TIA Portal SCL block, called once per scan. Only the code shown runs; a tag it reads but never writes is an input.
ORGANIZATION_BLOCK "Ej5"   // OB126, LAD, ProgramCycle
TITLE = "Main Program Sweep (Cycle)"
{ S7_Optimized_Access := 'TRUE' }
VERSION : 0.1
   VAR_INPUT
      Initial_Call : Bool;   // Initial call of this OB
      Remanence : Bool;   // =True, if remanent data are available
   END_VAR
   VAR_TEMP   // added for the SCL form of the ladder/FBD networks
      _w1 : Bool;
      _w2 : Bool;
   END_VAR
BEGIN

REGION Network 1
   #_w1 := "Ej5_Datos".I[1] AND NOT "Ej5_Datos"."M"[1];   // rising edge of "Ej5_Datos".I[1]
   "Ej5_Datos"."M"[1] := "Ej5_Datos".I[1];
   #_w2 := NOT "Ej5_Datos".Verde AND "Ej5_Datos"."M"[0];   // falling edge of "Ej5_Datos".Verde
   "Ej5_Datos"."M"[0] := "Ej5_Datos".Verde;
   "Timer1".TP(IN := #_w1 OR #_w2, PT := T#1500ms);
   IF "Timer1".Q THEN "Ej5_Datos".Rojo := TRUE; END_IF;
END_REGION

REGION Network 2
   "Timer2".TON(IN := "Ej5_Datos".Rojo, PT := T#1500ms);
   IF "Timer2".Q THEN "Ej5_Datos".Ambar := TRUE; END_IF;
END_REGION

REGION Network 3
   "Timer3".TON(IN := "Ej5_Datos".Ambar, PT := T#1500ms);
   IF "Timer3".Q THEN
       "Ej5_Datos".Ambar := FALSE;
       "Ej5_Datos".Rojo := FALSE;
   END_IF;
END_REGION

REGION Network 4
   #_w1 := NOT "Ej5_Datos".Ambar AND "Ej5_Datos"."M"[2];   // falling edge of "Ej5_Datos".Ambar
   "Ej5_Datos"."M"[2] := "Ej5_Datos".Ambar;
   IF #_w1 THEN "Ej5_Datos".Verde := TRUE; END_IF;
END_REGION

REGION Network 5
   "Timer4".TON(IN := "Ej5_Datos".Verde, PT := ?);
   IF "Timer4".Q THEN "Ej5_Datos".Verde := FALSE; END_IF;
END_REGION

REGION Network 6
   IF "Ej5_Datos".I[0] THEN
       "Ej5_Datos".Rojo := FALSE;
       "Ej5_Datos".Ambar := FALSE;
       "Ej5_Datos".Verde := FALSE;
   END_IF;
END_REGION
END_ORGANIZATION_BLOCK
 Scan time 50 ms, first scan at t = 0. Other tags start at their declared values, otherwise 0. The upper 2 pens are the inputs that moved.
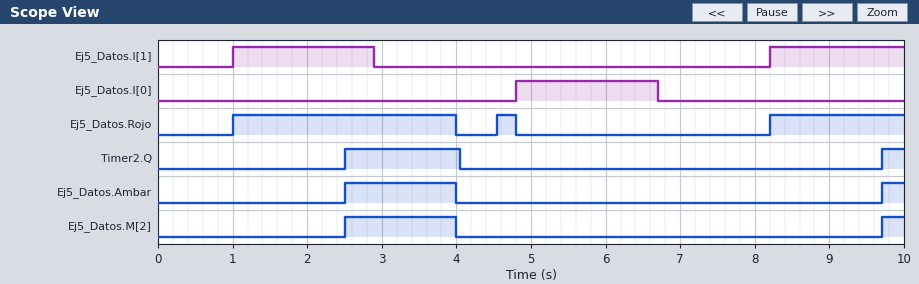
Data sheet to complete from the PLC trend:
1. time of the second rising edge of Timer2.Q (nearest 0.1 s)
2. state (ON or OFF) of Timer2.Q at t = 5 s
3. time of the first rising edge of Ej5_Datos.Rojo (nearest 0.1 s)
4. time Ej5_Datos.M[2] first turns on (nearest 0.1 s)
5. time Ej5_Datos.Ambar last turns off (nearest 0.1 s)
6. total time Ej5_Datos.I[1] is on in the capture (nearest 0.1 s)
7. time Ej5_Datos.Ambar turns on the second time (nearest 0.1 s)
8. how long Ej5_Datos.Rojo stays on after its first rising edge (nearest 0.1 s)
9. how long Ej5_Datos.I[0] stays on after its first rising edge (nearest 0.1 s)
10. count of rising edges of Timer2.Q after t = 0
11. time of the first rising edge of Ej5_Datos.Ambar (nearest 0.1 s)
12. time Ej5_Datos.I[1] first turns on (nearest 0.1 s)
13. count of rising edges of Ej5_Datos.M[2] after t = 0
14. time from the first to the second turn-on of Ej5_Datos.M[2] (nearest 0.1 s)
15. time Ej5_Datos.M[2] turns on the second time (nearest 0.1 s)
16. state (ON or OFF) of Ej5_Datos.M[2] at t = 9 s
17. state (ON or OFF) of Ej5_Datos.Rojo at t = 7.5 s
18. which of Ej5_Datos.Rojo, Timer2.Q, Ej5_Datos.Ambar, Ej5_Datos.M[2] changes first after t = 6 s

9.7 s
OFF
1.0 s
2.5 s
4.0 s
3.7 s
9.7 s
3.0 s
1.9 s
2
2.5 s
1.0 s
2
7.2 s
9.7 s
OFF
OFF
Ej5_Datos.Rojo
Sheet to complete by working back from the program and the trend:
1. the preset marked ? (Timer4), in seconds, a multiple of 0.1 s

0.5 s
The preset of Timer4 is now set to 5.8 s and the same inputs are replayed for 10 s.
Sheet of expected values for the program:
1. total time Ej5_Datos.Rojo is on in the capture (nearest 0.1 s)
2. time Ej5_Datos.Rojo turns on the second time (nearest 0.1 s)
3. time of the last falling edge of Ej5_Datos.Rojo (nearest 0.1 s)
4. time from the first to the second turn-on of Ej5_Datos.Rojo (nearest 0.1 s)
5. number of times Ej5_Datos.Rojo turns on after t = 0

4.8 s
8.2 s
4.0 s
7.2 s
2
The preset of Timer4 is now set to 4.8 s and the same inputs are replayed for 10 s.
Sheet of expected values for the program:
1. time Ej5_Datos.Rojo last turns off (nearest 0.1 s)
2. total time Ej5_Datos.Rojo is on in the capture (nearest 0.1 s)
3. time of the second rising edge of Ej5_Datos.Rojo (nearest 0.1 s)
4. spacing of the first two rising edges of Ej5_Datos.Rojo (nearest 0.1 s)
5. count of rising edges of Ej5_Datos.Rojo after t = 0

4.0 s
4.8 s
8.2 s
7.2 s
2
